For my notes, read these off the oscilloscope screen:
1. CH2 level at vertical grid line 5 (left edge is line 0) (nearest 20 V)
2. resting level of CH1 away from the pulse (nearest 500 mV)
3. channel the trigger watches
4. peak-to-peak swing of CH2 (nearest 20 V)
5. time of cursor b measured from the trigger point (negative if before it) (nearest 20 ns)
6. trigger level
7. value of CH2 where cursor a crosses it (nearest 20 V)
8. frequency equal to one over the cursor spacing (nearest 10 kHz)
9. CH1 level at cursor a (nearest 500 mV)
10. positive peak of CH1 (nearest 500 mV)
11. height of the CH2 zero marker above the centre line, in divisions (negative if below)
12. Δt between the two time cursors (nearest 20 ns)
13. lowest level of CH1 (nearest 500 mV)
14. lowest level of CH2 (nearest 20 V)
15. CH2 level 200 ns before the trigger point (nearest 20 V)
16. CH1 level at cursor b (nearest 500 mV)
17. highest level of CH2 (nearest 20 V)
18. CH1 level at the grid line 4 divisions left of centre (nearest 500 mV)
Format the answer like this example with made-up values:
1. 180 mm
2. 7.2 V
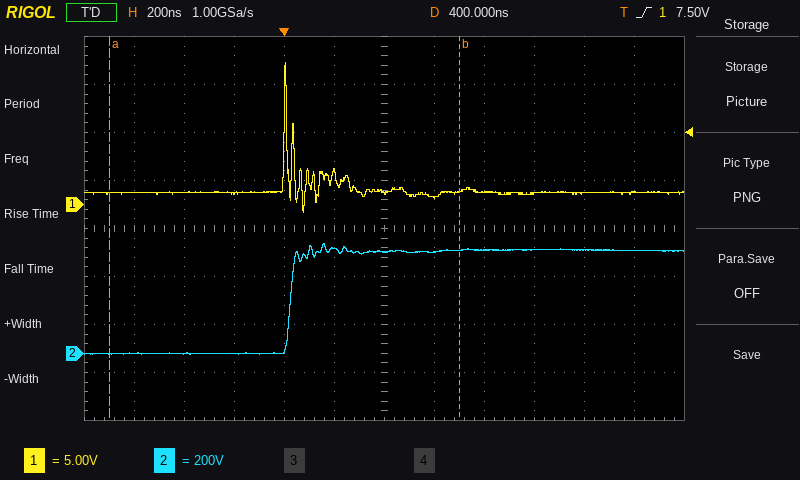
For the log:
1. 440 V
2. 1.0 V
3. CH1
4. 460 V
5. +700 ns
6. 7.50 V
7. 0 V
8. 710 kHz
9. 1.0 V
10. 15.0 V
11. -2.6 div
12. 1.40 µs
13. -1.0 V
14. 0 V
15. 0 V
16. 1.5 V
17. 460 V
18. 1.0 V
